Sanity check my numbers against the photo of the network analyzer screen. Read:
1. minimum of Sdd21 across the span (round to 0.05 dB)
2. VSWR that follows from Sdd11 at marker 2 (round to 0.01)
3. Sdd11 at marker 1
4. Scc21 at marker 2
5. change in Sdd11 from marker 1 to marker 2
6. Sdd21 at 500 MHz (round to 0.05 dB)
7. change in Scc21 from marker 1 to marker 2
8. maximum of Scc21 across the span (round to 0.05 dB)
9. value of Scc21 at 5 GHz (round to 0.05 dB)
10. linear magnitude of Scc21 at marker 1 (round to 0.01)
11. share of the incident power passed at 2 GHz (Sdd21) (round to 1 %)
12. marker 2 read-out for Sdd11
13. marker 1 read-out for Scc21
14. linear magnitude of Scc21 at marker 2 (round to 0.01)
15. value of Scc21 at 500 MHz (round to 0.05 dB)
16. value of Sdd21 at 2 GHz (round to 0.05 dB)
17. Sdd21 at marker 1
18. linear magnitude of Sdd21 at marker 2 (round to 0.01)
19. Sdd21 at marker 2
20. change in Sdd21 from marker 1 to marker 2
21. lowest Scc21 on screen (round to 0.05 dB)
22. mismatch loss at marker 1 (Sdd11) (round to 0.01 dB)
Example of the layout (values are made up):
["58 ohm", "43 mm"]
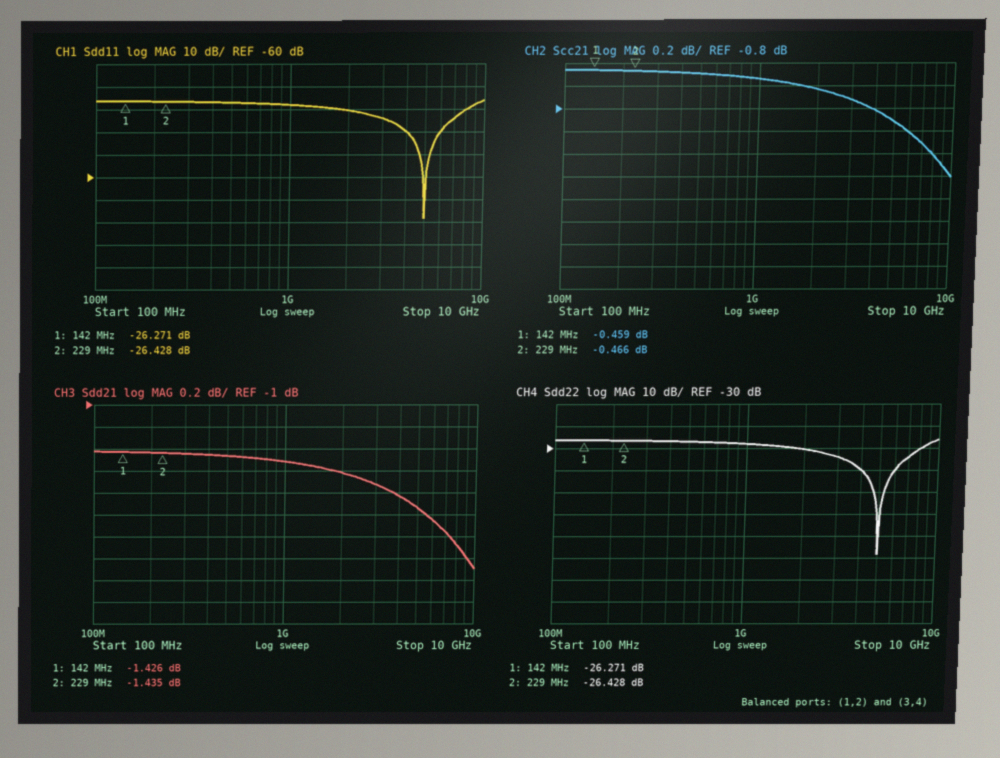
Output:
["-2.50 dB", "1.10", "-26.271 dB", "-0.466 dB", "-0.157 dB", "-1.45 dB", "-0.007 dB", "-0.45 dB", "-0.90 dB", "0.95", "69 %", "-26.428 dB", "-0.459 dB", "0.95", "-0.50 dB", "-1.60 dB", "-1.426 dB", "0.85", "-1.435 dB", "-0.009 dB", "-1.40 dB", "0.01 dB"]
